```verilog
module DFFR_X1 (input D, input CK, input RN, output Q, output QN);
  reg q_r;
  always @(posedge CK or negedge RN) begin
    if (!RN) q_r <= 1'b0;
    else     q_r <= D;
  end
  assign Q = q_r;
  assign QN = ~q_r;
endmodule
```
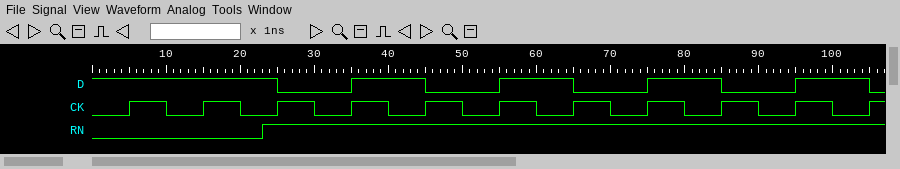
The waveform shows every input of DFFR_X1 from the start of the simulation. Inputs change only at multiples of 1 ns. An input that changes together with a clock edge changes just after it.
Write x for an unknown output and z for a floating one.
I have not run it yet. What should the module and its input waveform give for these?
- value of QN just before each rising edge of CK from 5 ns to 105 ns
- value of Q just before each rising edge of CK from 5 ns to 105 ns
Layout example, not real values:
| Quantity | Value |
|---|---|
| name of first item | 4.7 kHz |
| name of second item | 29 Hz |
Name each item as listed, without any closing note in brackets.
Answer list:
| Quantity | Value |
|---|---|
| value of QN just before each rising edge of CK from 5 ns to 105 ns | 1 1 1 0 1 0 1 0 1 0 1 |
| value of Q just before each rising edge of CK from 5 ns to 105 ns | 0 0 0 1 0 1 0 1 0 1 0 |
